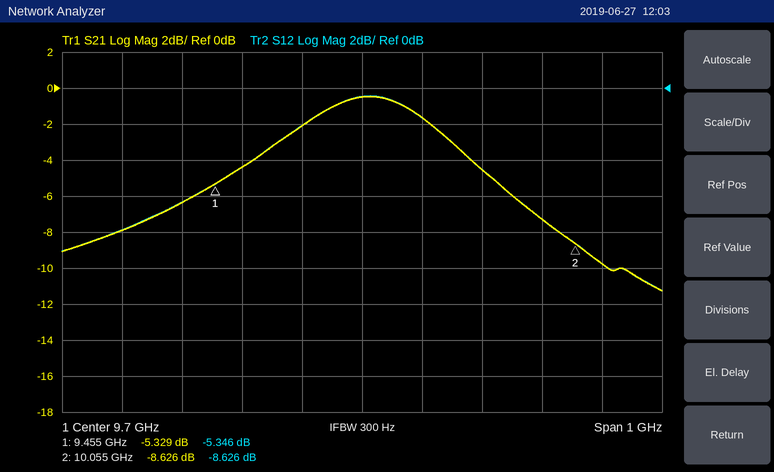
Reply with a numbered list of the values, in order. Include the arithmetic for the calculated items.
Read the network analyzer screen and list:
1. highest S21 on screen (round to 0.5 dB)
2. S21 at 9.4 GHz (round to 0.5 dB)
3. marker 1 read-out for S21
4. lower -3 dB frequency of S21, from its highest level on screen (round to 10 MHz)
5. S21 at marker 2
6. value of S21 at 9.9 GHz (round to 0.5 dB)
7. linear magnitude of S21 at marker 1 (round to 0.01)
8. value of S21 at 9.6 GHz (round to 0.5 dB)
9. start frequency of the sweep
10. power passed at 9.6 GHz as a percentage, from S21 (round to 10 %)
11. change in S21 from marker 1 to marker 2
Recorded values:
1. -0.5 dB
2. -6.5 dB
3. -5.329 dB
4. 9.54 GHz
5. -8.626 dB
6. -4.5 dB
7. 10^(-5.329/20) ≈ 0.54
8. -2.0 dB
9. 9.2 GHz
10. 10^(-2/10) ≈ 63.1 %, so 60 % to the nearest 10 %
11. -8.626 − (-5.329) = -3.297 dB
